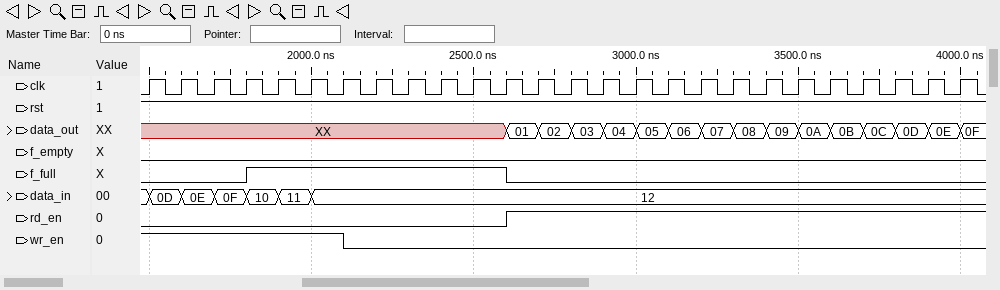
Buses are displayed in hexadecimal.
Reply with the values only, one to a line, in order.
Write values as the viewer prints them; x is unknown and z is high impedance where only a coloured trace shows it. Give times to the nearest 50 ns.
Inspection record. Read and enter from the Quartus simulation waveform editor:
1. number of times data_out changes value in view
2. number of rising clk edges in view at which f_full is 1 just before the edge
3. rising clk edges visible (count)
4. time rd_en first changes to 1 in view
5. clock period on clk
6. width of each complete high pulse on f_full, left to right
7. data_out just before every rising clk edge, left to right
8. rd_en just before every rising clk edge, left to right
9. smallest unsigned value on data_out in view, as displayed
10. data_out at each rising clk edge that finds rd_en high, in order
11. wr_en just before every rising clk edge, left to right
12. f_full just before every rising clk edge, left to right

15
8
26
2600 ns
100 ns
800 ns
XX, XX, XX, XX, XX, XX, XX, XX, XX, XX, XX, XX, 01, 02, 03, 04, 05, 06, 07, 08, 09, 0A, 0B, 0C, 0D, 0E
0 0 0 0 0 0 0 0 0 0 0 0 1 1 1 1 1 1 1 1 1 1 1 1 1 1
01
01, 02, 03, 04, 05, 06, 07, 08, 09, 0A, 0B, 0C, 0D, 0E
1 1 1 1 1 1 1 0 0 0 0 0 0 0 0 0 0 0 0 0 0 0 0 0 0 0
0 0 0 0 1 1 1 1 1 1 1 1 0 0 0 0 0 0 0 0 0 0 0 0 0 0
